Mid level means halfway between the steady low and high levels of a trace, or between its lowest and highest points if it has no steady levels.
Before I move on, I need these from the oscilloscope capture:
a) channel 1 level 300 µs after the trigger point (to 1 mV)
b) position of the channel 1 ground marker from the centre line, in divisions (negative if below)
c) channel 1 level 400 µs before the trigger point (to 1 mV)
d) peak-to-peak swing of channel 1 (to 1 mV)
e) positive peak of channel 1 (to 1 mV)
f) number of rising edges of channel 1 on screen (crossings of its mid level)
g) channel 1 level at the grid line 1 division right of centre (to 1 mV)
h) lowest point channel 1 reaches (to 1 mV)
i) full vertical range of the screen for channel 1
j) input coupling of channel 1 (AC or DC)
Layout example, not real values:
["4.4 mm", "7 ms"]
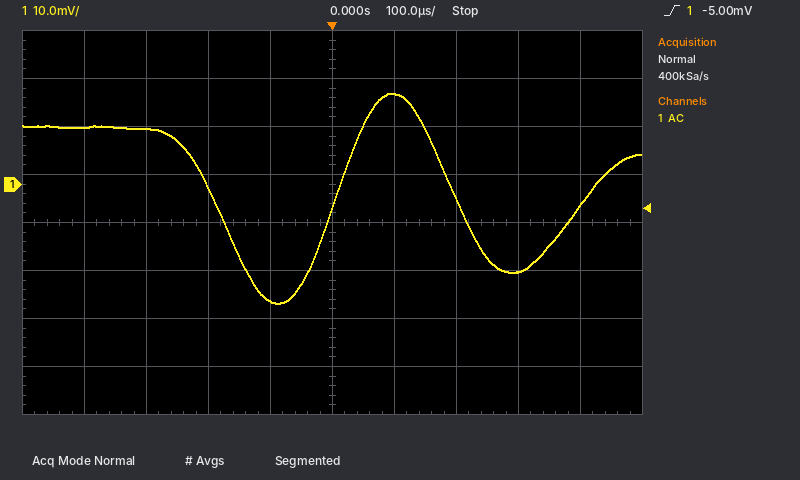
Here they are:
["-18 mV", "+0.8 div", "12 mV", "44 mV", "19 mV", "2", "19 mV", "-25 mV", "80 mV", "AC"]
